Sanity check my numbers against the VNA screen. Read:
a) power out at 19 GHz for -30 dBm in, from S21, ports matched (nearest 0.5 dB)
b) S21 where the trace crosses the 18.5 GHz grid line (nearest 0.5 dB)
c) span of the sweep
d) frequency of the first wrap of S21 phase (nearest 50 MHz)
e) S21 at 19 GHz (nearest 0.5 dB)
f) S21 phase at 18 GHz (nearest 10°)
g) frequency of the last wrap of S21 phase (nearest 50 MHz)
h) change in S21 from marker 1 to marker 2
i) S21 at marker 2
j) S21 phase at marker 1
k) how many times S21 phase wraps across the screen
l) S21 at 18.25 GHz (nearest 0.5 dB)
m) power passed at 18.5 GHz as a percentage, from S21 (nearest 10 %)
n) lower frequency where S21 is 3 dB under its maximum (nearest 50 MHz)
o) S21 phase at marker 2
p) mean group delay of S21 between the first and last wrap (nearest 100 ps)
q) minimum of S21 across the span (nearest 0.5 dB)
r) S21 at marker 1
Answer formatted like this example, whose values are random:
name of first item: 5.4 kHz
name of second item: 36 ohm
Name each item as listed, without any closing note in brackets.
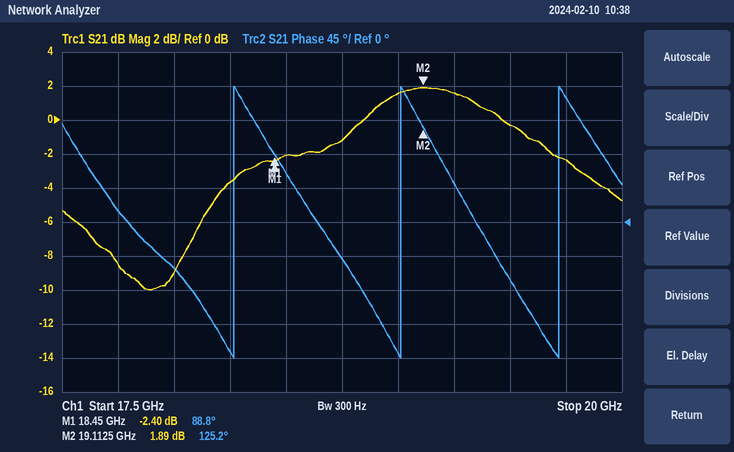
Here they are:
power out at 19 GHz for -30 dBm in, from S21, ports matched: -28.5 dBm
S21 where the trace crosses the 18.5 GHz grid line: -2.0 dB
span of the sweep: 2.5 GHz
frequency of the first wrap of S21 phase: 18.25 GHz
S21 at 19 GHz: 1.5 dB
S21 phase at 18 GHz: -60°
frequency of the last wrap of S21 phase: 19.70 GHz
change in S21 from marker 1 to marker 2: 4.29 dB
S21 at marker 2: 1.89 dB
S21 phase at marker 1: 88.8°
how many times S21 phase wraps across the screen: 3
S21 at 18.25 GHz: -3.5 dB
power passed at 18.5 GHz as a percentage, from S21: 60 %
lower frequency where S21 is 3 dB under its maximum: 18.75 GHz
S21 phase at marker 2: 125.2°
mean group delay of S21 between the first and last wrap: 1.4 ns
minimum of S21 across the span: -10.0 dB
S21 at marker 1: -2.40 dB
